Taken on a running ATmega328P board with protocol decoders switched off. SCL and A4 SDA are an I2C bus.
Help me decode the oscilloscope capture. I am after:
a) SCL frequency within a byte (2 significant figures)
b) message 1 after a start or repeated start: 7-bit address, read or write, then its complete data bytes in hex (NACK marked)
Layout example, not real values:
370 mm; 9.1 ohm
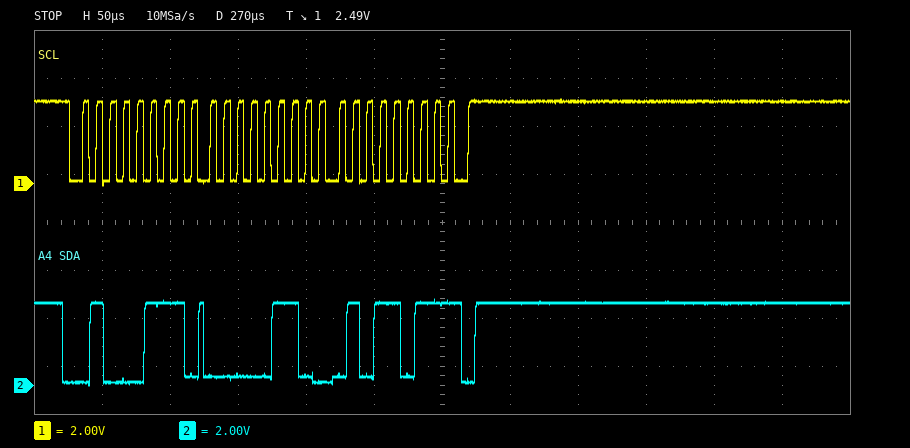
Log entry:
100 kHz; 0x23 read: 06 5B NACK
